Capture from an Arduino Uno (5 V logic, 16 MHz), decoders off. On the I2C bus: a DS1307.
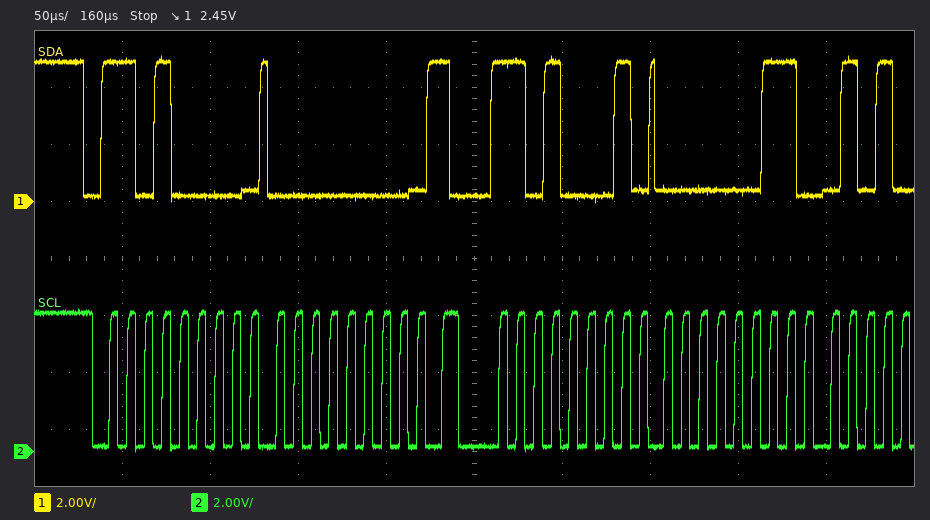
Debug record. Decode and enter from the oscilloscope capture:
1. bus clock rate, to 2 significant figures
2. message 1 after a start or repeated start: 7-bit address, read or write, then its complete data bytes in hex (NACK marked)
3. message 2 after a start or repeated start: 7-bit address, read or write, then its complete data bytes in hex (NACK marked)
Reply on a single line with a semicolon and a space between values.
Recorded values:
100 kHz; 0x68 write: 00; 0x68 read: 03
